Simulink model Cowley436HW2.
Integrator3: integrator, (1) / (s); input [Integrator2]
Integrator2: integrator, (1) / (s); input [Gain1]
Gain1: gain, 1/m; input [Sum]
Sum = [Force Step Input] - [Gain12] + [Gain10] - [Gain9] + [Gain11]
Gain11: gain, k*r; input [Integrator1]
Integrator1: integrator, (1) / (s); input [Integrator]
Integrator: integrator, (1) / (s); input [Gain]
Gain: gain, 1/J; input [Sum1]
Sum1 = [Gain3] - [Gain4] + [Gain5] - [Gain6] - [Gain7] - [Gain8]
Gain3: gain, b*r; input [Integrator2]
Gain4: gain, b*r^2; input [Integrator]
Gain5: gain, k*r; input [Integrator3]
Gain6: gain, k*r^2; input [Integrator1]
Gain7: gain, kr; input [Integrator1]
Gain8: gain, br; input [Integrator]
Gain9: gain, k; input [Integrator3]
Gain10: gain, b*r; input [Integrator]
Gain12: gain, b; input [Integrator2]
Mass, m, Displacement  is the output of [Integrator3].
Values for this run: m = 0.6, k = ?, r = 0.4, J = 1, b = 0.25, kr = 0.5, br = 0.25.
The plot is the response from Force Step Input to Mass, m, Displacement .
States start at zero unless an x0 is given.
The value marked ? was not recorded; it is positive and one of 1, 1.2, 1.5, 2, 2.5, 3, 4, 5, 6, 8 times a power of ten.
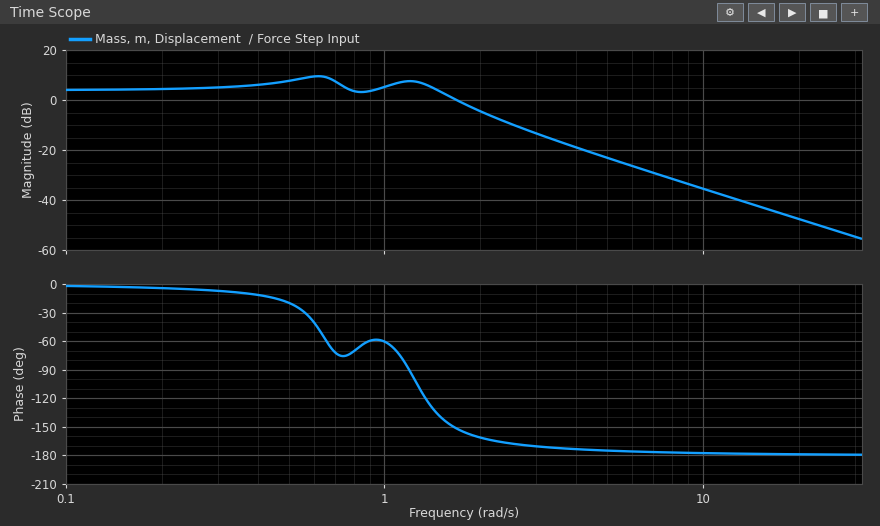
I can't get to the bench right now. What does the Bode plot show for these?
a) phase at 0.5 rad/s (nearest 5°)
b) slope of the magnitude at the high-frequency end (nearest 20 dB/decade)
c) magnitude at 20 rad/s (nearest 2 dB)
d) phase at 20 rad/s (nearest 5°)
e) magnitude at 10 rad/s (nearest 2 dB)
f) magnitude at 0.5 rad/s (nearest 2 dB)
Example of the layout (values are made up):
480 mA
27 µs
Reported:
-20°
-40 dB/decade
-48 dB
-180°
-36 dB
8 dB
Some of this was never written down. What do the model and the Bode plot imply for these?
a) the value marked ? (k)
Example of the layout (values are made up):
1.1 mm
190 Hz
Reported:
0.8
